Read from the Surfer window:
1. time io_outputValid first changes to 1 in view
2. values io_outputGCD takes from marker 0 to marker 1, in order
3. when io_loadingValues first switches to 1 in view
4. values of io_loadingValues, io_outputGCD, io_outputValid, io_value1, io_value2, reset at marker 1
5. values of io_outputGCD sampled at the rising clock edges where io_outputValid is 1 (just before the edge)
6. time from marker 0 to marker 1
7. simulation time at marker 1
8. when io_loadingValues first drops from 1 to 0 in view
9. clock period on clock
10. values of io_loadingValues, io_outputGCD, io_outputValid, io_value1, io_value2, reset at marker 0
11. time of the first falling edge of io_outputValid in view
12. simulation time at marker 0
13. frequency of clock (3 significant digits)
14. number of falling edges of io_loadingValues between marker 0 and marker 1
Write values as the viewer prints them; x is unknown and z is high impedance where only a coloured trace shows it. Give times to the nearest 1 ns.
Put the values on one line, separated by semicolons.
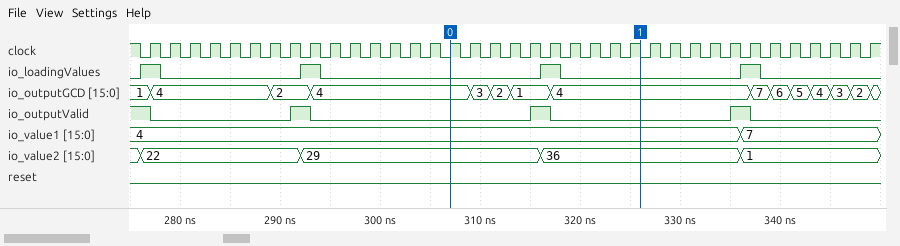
291 ns; 4, 3, 2, 1, 4; 276 ns; io_loadingValues=0, io_outputGCD=4, io_outputValid=0, io_value1=4, io_value2=36, reset=0; 1, 2, 1, 4; 19 ns; 326 ns; 278 ns; 2 ns; io_loadingValues=0, io_outputGCD=4, io_outputValid=0, io_value1=4, io_value2=29, reset=0; 277 ns; 307 ns; 500 MHz; 1
